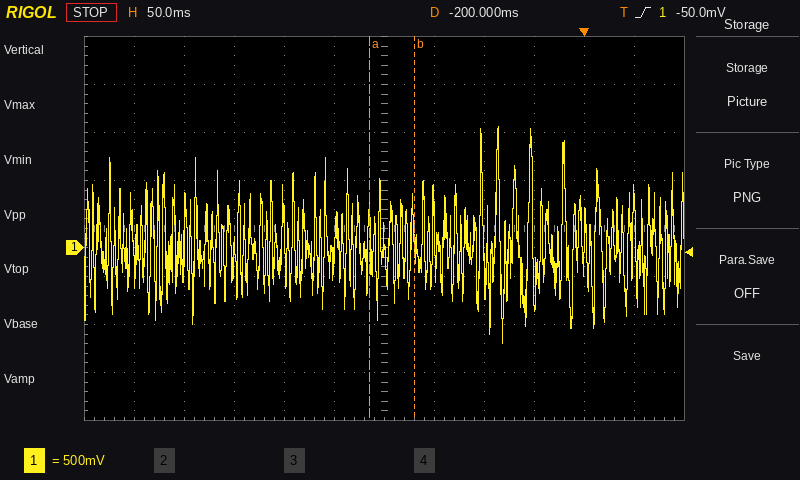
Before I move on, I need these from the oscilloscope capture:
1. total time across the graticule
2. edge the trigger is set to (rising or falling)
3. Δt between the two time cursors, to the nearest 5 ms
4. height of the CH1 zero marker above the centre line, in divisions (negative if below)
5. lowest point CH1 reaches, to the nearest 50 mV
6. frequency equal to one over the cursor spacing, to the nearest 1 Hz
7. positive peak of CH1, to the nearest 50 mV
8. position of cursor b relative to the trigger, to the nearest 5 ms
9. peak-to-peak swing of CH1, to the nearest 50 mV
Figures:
600 ms
rising
45 ms
-0.4 div
-1.00 V
22 Hz
1.25 V
-170 ms
2.25 V
